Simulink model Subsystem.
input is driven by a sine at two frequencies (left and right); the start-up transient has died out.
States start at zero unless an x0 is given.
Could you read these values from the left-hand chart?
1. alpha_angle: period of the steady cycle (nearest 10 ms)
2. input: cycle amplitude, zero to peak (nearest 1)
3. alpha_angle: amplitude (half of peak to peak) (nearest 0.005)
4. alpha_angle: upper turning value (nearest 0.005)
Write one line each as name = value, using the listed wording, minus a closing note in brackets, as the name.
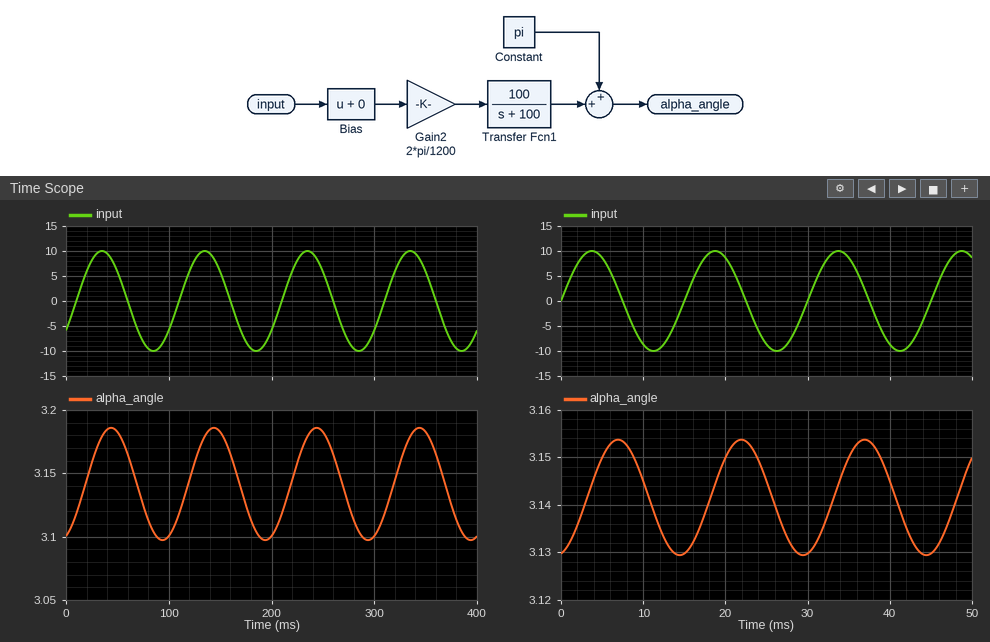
alpha_angle: period of the steady cycle = 100 ms
input: cycle amplitude, zero to peak = 10
alpha_angle: amplitude (half of peak to peak) = 0.045
alpha_angle: upper turning value = 3.185
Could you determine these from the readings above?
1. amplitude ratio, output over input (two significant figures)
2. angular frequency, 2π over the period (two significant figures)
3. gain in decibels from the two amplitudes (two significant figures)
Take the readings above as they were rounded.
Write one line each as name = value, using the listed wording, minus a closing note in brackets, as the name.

amplitude ratio, output over input = 0.0045
angular frequency, 2π over the period = 0.063 rad/ms
gain in decibels from the two amplitudes = -47 dB
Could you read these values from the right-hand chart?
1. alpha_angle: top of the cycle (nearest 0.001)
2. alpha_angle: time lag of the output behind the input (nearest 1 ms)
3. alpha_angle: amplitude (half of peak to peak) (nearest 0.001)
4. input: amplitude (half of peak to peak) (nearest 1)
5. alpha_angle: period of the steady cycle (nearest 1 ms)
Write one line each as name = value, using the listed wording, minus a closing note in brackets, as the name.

alpha_angle: top of the cycle = 3.154
alpha_angle: time lag of the output behind the input = 3 ms
alpha_angle: amplitude (half of peak to peak) = 0.012
input: amplitude (half of peak to peak) = 10
alpha_angle: period of the steady cycle = 15 ms
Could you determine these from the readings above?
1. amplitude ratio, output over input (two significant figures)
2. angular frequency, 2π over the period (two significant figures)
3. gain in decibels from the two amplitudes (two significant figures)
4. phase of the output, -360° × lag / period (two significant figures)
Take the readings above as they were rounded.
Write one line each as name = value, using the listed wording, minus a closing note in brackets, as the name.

amplitude ratio, output over input = 0.0012
angular frequency, 2π over the period = 0.42 rad/ms
gain in decibels from the two amplitudes = -58 dB
phase of the output, -360° × lag / period = -72°
